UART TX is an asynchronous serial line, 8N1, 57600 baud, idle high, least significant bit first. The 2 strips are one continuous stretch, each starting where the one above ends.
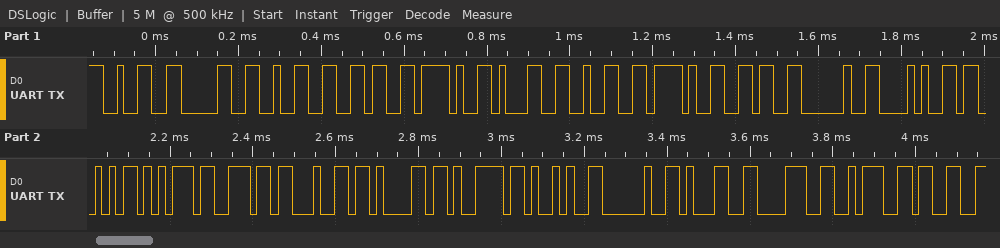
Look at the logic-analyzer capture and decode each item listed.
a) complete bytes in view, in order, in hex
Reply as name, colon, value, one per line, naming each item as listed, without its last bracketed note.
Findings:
complete bytes in view, in order, in hex: 0x32 0x30 0x32 0x36 0x2F 0x31 0x32 0x2F 0x36 0x20 0x28 0x53 0x75 0x6E 0x64 0x61 0x79 0x29 0x20 0x31 0x38 0x3A 0x33
